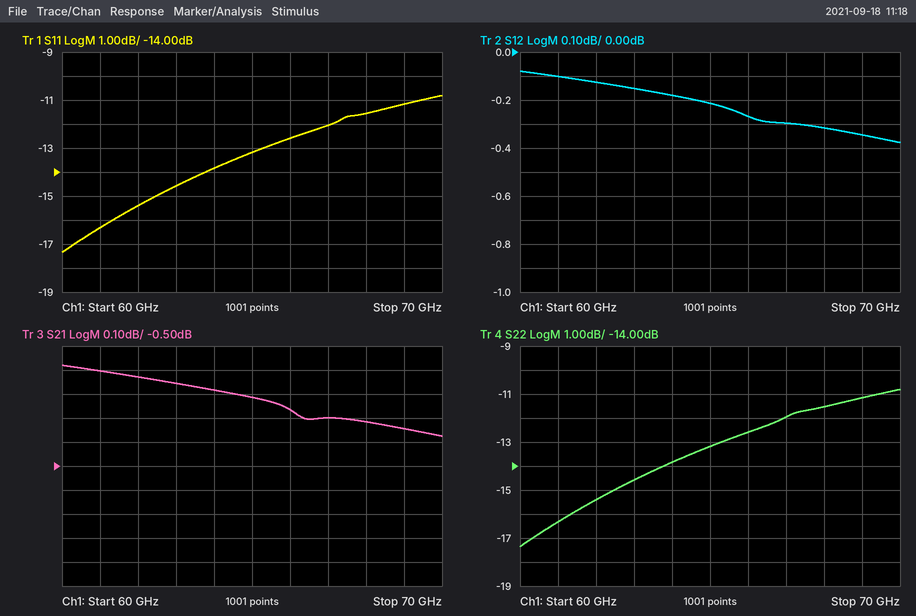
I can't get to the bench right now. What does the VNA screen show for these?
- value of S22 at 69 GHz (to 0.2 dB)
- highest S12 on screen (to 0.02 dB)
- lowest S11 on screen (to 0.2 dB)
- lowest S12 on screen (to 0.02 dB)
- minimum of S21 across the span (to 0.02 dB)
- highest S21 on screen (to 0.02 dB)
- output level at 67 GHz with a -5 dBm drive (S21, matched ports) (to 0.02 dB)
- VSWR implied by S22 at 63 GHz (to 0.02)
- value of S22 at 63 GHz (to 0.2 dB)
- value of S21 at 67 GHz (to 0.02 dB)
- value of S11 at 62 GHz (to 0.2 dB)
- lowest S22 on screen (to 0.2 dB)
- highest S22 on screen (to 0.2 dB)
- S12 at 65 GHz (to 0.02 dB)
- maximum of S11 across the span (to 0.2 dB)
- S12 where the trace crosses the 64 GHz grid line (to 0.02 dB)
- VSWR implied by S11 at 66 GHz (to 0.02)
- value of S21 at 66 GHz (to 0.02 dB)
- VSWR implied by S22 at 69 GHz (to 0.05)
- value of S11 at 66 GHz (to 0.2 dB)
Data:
-11.2 dB
-0.08 dB
-17.4 dB
-0.38 dB
-0.38 dB
-0.08 dB
-5.30 dBm
1.46
-14.6 dB
-0.30 dB
-15.4 dB
-17.4 dB
-10.8 dB
-0.22 dB
-10.8 dB
-0.18 dB
1.62
-0.26 dB
1.75
-12.6 dB
